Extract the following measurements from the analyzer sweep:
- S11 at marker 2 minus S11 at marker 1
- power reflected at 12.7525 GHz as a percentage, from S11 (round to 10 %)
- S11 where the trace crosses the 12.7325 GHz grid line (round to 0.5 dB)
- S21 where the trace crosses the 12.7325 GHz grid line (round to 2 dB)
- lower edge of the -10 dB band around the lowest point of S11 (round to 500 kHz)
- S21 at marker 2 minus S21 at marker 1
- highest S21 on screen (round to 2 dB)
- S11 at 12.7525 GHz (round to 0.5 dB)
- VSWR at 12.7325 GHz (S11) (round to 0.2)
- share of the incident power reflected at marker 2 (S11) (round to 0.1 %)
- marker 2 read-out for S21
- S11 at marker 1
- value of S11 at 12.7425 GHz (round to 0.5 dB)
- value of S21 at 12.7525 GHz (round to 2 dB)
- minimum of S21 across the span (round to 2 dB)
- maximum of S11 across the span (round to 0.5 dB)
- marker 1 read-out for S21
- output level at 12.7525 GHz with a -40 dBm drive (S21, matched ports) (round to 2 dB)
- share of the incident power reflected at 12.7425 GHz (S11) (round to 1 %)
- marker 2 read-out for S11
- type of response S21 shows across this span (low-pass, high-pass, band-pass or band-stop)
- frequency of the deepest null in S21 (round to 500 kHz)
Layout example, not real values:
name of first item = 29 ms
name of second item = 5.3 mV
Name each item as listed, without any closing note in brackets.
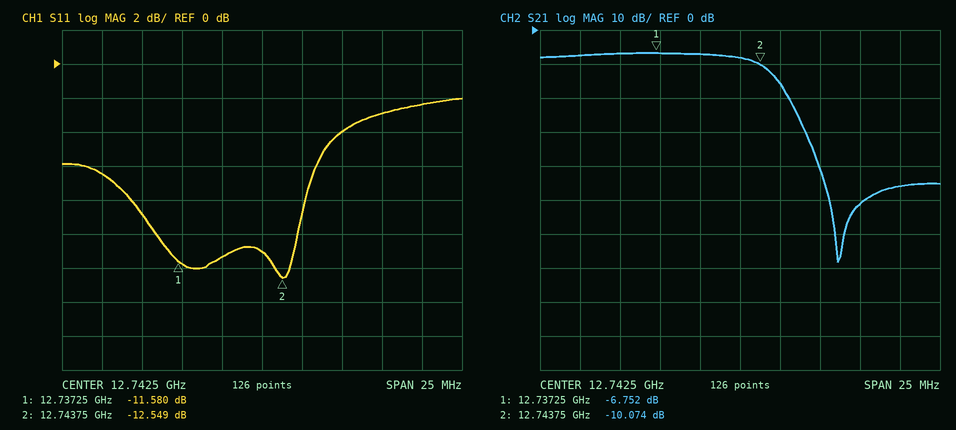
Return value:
S11 at marker 2 minus S11 at marker 1 = -0.969 dB
power reflected at 12.7525 GHz as a percentage, from S11 = 60 %
S11 where the trace crosses the 12.7325 GHz grid line = -6.5 dB
S21 where the trace crosses the 12.7325 GHz grid line = -8 dB
lower edge of the -10 dB band around the lowest point of S11 = 12.7360 GHz
S21 at marker 2 minus S21 at marker 1 = -3.322 dB
highest S21 on screen = -6 dB
S11 at 12.7525 GHz = -2.5 dB
VSWR at 12.7325 GHz (S11) = 2.8
share of the incident power reflected at marker 2 (S11) = 5.6 %
marker 2 read-out for S21 = -10.074 dB
S11 at marker 1 = -11.580 dB
value of S11 at 12.7425 GHz = -11.0 dB
value of S21 at 12.7525 GHz = -46 dB
minimum of S21 across the span = -68 dB
maximum of S11 across the span = -2.0 dB
marker 1 read-out for S21 = -6.752 dB
output level at 12.7525 GHz with a -40 dBm drive (S21, matched ports) = -86 dBm
share of the incident power reflected at 12.7425 GHz (S11) = 8 %
marker 2 read-out for S11 = -12.549 dB
type of response S21 shows across this span = low-pass
frequency of the deepest null in S21 = 12.7485 GHz
